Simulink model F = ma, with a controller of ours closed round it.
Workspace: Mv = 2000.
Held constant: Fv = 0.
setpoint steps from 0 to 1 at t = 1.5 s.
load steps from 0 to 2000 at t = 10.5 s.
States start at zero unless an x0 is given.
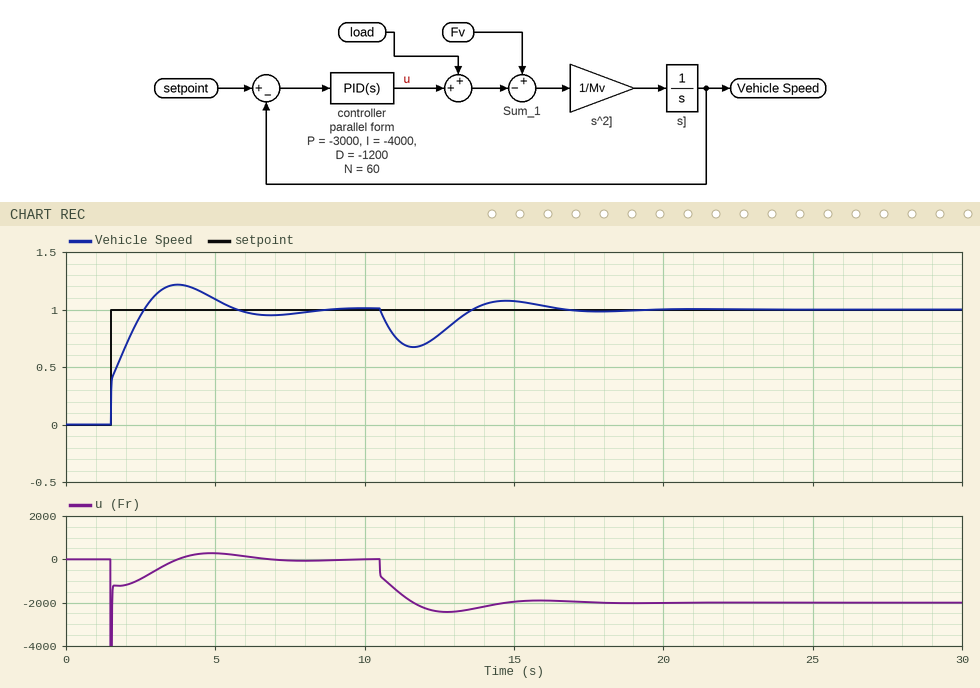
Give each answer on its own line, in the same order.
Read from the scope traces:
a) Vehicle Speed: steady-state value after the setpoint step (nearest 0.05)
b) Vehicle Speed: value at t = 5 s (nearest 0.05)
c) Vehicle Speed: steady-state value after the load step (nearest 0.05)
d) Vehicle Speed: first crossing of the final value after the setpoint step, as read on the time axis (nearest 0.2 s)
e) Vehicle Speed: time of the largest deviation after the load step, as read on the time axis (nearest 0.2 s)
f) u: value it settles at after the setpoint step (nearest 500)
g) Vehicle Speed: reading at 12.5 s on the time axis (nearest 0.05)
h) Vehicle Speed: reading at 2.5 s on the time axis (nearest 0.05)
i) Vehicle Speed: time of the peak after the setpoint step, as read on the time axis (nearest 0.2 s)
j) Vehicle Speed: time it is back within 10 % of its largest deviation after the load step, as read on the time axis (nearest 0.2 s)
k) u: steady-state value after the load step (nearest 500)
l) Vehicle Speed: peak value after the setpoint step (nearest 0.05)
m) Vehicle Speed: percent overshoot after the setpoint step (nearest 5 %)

1.00
1.10
1.00
2.6 s
11.6 s
0
0.80
0.95
3.8 s
16.0 s
-2000
1.20
20 %
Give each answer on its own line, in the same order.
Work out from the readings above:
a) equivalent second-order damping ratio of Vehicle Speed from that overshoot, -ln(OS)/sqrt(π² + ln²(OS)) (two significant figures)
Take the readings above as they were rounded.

0.46
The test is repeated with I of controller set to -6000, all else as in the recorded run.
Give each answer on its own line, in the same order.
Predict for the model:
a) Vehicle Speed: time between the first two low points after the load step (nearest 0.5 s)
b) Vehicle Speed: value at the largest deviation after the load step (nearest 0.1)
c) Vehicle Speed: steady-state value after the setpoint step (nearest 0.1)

5.0 s
0.7
1.0
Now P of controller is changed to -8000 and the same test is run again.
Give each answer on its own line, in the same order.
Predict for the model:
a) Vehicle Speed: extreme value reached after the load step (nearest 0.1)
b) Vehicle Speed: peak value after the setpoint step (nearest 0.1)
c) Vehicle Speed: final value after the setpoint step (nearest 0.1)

0.8
1.1
1.0
